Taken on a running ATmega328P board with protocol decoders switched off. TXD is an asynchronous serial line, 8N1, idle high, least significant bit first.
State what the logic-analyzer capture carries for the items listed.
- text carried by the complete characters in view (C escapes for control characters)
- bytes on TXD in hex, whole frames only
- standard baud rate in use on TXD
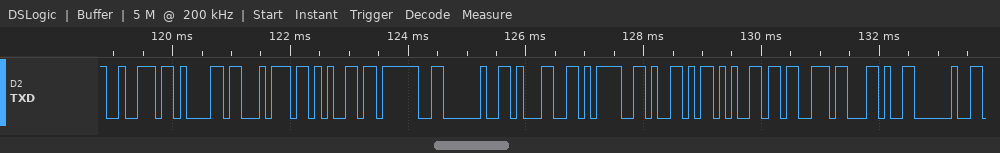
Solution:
"rate? 1=Yes, "
72 61 74 65 3F 20 31 3D 59 65 73 2C 20
9600 baud
